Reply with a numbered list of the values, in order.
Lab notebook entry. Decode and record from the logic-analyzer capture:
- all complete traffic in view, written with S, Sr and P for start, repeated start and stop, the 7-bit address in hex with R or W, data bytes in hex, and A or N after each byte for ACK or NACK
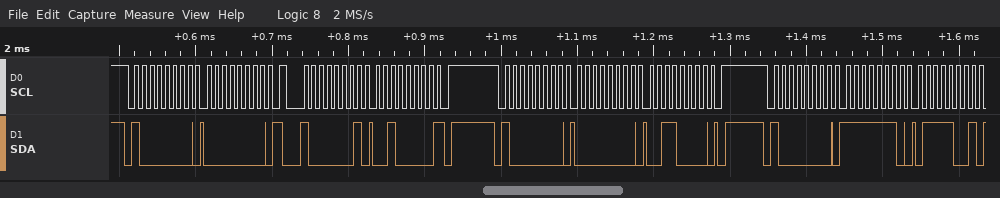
1. S 40W A 00 A Sr 40R A 20 N P S 40W A 00 A 30 A P S 40W A FE A 79 A
